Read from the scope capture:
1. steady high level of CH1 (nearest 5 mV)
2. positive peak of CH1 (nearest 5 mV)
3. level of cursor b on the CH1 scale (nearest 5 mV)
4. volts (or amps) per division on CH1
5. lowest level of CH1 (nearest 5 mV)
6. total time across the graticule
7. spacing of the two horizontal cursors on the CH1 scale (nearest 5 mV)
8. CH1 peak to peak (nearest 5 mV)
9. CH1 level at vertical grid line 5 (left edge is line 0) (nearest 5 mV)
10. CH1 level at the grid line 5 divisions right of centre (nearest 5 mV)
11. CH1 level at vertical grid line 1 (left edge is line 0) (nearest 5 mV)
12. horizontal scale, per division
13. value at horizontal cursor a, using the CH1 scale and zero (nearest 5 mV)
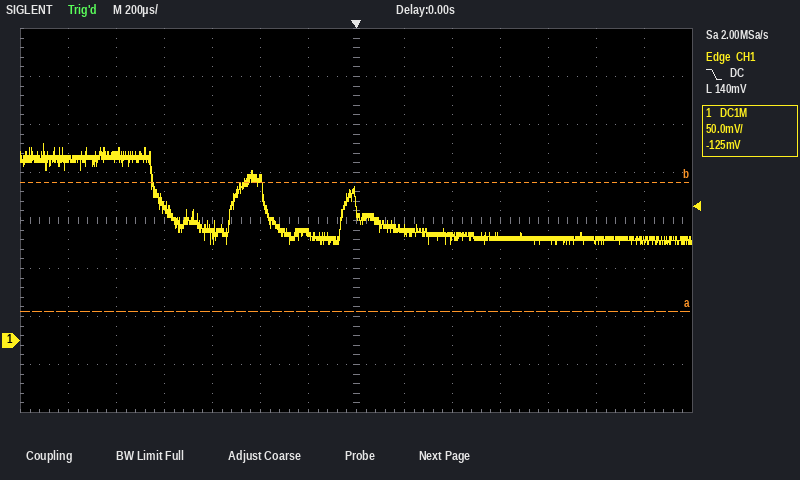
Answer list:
190 mV
205 mV
165 mV
50 mV
100 mV
2.8 ms
135 mV
105 mV
170 mV
105 mV
190 mV
200 µs
30 mV
